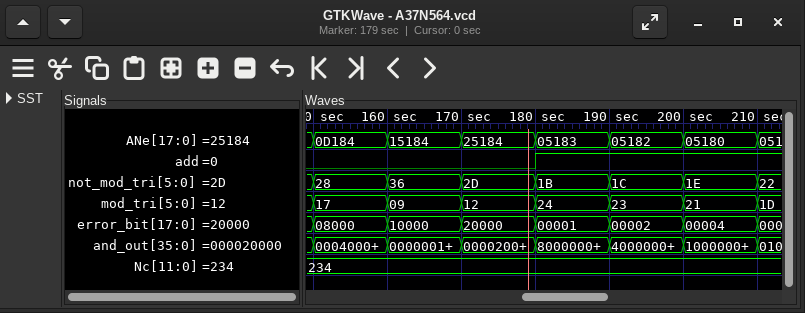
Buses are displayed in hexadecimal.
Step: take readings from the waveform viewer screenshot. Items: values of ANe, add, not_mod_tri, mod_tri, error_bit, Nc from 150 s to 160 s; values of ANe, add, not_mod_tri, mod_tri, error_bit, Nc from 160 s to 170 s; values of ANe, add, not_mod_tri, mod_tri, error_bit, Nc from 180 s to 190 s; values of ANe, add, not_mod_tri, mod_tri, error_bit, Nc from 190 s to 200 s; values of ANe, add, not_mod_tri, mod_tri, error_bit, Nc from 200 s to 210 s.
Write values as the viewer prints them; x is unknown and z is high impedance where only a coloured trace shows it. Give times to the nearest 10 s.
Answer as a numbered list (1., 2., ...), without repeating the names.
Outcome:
1. ANe=0D184, add=0, not_mod_tri=28, mod_tri=17, error_bit=08000, Nc=234
2. ANe=15184, add=0, not_mod_tri=36, mod_tri=09, error_bit=10000, Nc=234
3. ANe=05183, add=1, not_mod_tri=1B, mod_tri=24, error_bit=00001, Nc=234
4. ANe=05182, add=1, not_mod_tri=1C, mod_tri=23, error_bit=00002, Nc=234
5. ANe=05180, add=1, not_mod_tri=1E, mod_tri=21, error_bit=00004, Nc=234
